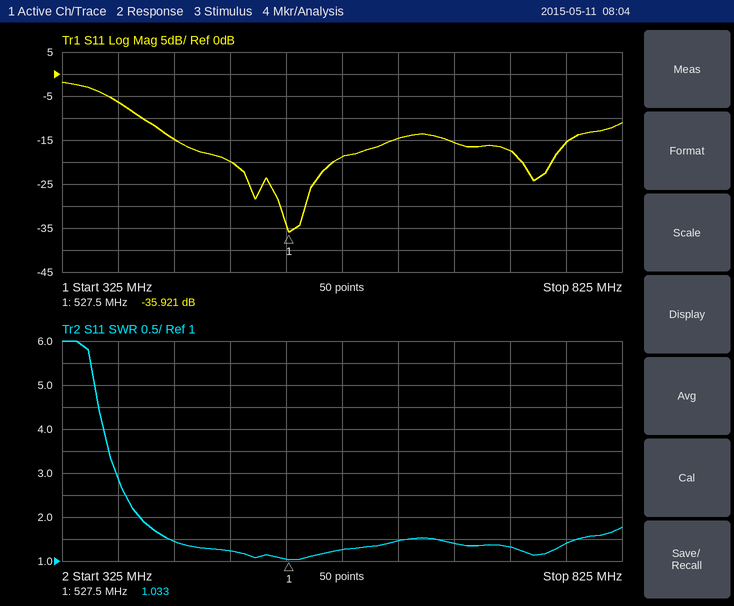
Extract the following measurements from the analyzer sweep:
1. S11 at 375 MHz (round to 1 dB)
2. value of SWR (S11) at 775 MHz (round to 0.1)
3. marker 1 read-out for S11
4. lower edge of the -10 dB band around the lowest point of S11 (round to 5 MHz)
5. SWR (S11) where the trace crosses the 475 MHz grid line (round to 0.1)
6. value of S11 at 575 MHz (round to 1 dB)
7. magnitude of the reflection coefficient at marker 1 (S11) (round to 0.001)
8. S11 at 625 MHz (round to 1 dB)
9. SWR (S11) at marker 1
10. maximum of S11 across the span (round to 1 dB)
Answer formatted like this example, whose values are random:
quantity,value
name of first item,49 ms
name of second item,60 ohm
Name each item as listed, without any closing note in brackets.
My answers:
quantity,value
S11 at 375 MHz,-6 dB
value of SWR (S11) at 775 MHz,1.4
marker 1 read-out for S11,-35.921 dB
lower edge of the -10 dB band around the lowest point of S11,395 MHz
SWR (S11) where the trace crosses the 475 MHz grid line,1.2
value of S11 at 575 MHz,-19 dB
magnitude of the reflection coefficient at marker 1 (S11),0.016
S11 at 625 MHz,-15 dB
SWR (S11) at marker 1,1.033
maximum of S11 across the span,-2 dB
